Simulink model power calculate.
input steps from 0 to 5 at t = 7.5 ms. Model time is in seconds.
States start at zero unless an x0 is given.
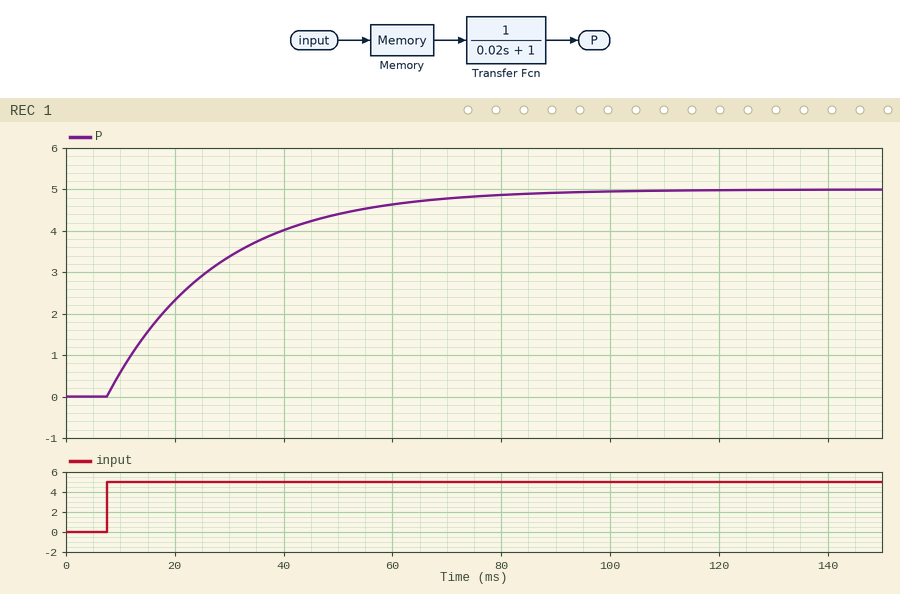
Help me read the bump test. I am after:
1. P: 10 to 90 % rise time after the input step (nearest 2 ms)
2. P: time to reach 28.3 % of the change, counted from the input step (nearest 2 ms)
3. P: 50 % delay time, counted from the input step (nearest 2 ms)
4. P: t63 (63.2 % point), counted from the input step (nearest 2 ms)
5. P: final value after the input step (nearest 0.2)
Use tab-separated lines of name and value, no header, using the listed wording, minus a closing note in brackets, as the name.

P: 10 to 90 % rise time after the input step	44 ms
P: time to reach 28.3 % of the change, counted from the input step	6 ms
P: 50 % delay time, counted from the input step	14 ms
P: t63 (63.2 % point), counted from the input step	20 ms
P: final value after the input step	5.0
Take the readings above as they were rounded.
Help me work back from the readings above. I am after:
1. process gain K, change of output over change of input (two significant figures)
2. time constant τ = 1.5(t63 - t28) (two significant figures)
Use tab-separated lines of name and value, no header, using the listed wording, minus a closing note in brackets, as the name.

process gain K, change of output over change of input	1.0
time constant τ = 1.5(t63 - t28)	21 ms
